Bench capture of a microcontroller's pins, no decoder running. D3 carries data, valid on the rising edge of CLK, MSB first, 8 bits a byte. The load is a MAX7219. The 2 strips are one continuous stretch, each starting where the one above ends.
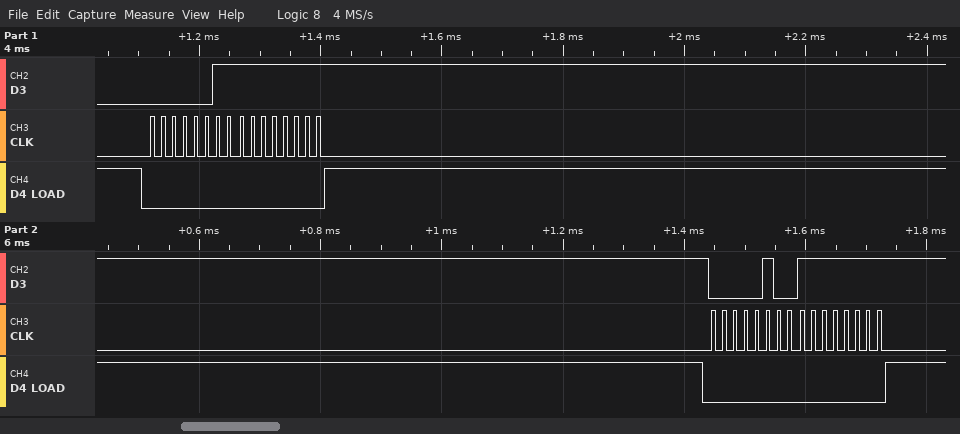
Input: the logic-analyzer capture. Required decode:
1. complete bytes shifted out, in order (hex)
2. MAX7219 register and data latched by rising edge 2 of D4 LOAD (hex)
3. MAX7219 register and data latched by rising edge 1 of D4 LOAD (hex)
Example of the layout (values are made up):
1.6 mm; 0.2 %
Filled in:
03 FF 04 FF; register 0x4, data 0xFF; register 0x3, data 0xFF
